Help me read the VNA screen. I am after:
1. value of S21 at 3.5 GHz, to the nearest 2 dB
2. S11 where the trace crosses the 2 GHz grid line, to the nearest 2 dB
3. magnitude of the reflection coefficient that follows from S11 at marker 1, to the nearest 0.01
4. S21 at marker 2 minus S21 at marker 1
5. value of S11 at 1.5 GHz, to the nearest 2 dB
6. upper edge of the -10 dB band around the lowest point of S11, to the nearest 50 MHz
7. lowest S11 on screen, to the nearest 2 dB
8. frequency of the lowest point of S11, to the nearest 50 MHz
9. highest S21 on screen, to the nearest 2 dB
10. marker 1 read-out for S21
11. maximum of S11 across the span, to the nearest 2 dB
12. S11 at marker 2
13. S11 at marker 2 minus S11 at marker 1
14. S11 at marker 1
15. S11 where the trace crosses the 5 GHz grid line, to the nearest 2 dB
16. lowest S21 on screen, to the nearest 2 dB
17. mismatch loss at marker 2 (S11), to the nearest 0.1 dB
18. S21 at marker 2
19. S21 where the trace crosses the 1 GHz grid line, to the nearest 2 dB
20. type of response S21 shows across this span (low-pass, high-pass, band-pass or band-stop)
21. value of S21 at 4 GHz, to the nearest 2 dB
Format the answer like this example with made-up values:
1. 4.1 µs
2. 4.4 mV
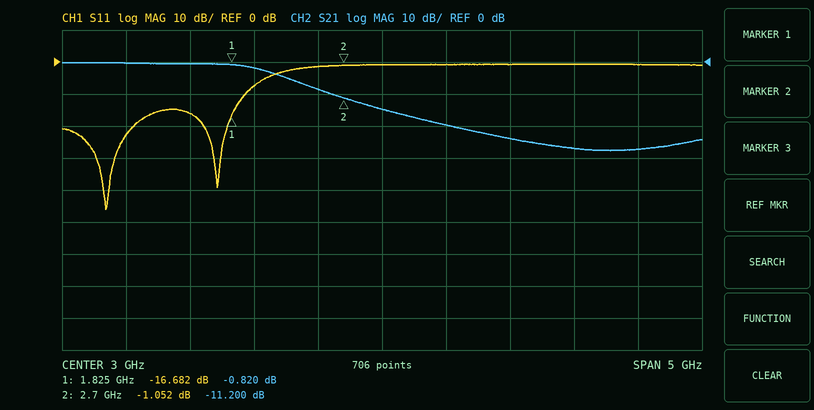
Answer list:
1. -20 dB
2. -8 dB
3. 0.15
4. -10.380 dB
5. -16 dB
6. 1.95 GHz
7. -46 dB
8. 850 MHz
9. 0 dB
10. -0.820 dB
11. 0 dB
12. -1.052 dB
13. 15.630 dB
14. -16.682 dB
15. 0 dB
16. -28 dB
17. 6.7 dB
18. -11.200 dB
19. 0 dB
20. low-pass
21. -24 dB
